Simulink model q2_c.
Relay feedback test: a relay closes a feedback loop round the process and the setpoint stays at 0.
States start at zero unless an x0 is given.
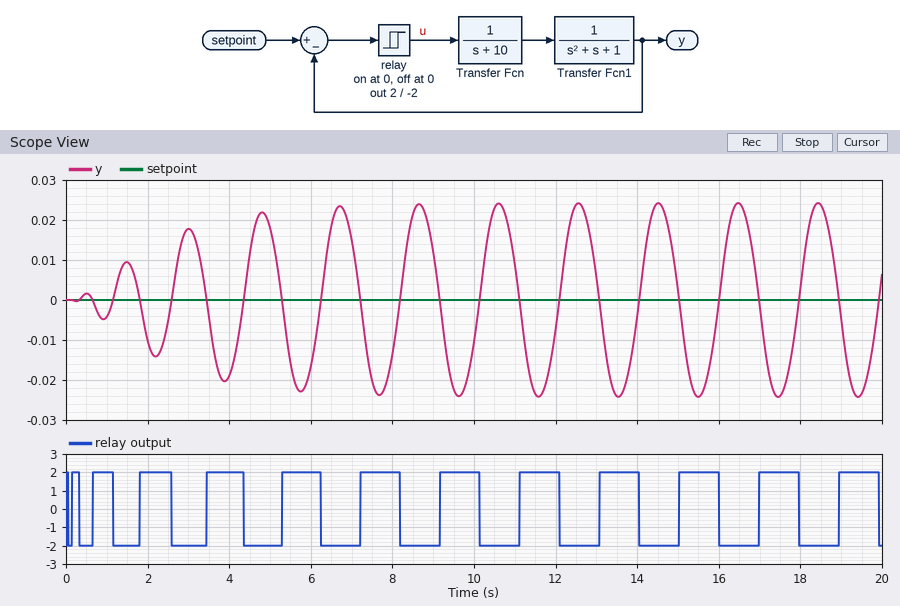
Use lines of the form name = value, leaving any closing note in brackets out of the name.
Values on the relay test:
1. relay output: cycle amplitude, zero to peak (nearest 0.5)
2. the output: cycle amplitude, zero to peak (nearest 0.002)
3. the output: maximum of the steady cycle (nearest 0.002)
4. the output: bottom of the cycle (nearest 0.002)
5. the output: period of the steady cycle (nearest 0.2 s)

relay output: cycle amplitude, zero to peak = 2.0
the output: cycle amplitude, zero to peak = 0.024
the output: maximum of the steady cycle = 0.024
the output: bottom of the cycle = -0.024
the output: period of the steady cycle = 2.0 s
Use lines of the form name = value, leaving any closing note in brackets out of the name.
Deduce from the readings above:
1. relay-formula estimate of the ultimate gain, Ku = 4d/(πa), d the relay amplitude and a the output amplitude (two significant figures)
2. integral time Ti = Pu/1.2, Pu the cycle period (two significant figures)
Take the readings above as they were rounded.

relay-formula estimate of the ultimate gain, Ku = 4d/(πa), d the relay amplitude and a the output amplitude = 110
integral time Ti = Pu/1.2, Pu the cycle period = 1.7 s
